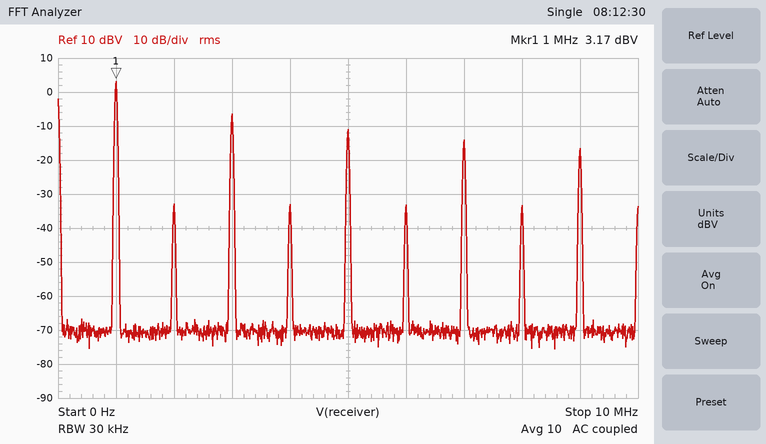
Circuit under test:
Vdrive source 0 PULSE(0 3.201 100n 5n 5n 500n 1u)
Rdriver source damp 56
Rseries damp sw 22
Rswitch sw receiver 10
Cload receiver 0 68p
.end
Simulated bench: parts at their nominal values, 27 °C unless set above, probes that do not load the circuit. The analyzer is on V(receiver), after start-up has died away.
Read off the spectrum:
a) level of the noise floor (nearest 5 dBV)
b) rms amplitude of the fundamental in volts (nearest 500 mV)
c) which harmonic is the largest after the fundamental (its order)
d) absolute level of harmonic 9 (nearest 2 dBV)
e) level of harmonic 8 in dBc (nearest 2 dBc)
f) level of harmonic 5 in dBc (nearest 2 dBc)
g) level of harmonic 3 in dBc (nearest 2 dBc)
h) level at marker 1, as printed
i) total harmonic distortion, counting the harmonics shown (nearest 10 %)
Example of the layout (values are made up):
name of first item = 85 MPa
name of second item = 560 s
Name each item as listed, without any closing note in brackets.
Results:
level of the noise floor = -70 dBV
rms amplitude of the fundamental in volts = 1.5 V
which harmonic is the largest after the fundamental = 3
absolute level of harmonic 9 = -16 dBV
level of harmonic 8 in dBc = -36 dBc
level of harmonic 5 in dBc = -14 dBc
level of harmonic 3 in dBc = -10 dBc
level at marker 1, as printed = 3.17 dBV
total harmonic distortion, counting the harmonics shown = 40 %
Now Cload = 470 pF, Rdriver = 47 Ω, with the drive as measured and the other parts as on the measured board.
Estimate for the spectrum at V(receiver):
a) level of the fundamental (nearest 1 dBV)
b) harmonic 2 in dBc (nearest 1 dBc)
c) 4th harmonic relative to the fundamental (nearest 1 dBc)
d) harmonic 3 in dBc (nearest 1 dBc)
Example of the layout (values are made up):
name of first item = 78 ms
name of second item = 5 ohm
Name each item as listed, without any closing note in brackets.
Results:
level of the fundamental = 3 dBV
harmonic 2 in dBc = -37 dBc
4th harmonic relative to the fundamental = -39 dBc
harmonic 3 in dBc = -11 dBc
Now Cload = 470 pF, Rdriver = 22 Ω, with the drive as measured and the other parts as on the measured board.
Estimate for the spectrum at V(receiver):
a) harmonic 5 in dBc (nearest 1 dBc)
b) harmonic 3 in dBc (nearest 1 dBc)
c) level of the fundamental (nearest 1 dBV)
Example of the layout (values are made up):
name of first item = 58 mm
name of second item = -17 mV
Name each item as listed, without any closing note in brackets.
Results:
harmonic 5 in dBc = -16 dBc
harmonic 3 in dBc = -10 dBc
level of the fundamental = 3 dBV
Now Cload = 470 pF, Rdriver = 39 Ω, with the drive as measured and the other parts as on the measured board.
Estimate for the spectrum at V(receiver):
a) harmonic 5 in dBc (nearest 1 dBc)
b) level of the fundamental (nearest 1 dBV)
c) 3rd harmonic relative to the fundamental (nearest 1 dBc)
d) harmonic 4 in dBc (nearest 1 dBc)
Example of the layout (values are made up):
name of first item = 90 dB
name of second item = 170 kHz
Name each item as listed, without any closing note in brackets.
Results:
harmonic 5 in dBc = -17 dBc
level of the fundamental = 3 dBV
3rd harmonic relative to the fundamental = -11 dBc
harmonic 4 in dBc = -38 dBc
